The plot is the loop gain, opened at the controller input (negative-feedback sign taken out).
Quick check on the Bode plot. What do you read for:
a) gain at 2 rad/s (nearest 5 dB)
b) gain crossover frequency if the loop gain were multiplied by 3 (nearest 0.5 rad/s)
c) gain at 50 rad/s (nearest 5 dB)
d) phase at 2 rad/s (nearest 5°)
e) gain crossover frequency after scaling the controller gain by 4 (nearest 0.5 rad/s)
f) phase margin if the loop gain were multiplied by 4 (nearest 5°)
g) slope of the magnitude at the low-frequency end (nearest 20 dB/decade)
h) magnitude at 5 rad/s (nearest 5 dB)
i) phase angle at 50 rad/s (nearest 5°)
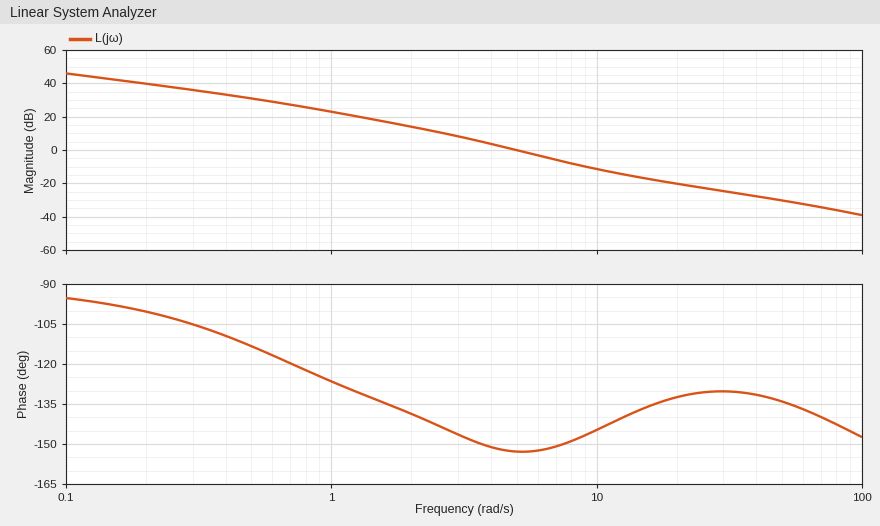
15 dB
9.0 rad/s
-30 dB
-140°
10.5 rad/s
35°
-20 dB/decade
0 dB
-135°
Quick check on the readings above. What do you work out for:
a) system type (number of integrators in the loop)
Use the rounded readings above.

1
